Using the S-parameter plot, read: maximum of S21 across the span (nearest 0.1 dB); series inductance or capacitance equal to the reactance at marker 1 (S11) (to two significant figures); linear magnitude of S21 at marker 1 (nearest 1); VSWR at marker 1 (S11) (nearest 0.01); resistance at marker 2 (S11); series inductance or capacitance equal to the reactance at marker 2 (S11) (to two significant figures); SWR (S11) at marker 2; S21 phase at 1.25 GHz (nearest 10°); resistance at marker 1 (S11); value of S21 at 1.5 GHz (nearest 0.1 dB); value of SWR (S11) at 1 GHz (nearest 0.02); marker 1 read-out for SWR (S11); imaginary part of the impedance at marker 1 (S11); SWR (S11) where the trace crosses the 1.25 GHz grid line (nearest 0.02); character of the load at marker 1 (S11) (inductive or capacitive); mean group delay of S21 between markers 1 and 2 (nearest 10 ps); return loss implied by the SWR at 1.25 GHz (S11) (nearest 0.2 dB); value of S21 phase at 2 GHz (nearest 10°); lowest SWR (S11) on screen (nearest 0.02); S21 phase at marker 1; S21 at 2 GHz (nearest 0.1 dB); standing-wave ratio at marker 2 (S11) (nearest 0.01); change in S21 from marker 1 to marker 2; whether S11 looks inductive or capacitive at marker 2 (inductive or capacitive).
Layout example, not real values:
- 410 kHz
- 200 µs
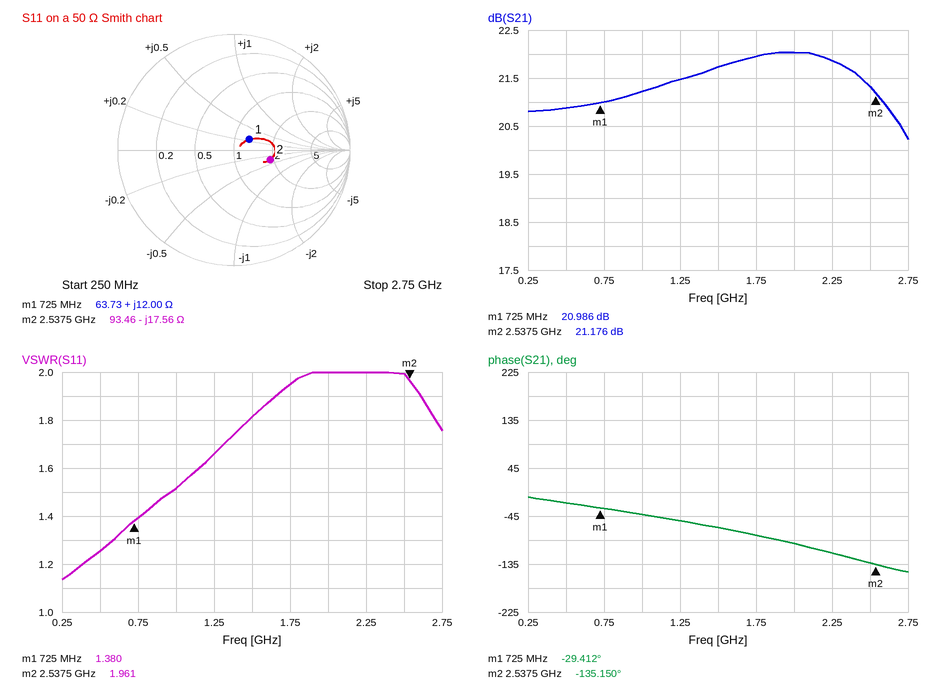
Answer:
- 22.0 dB
- 2.6 nH
- 11
- 1.38
- 93.46 Ω
- 3.6 pF
- 1.961
- -50°
- 63.73 Ω
- 21.7 dB
- 1.52
- 1.380
- +12.00 Ω
- 1.66
- inductive
- 160 ps
- 12.2 dB
- -100°
- 1.14
- -29.412°
- 22.0 dB
- 1.96
- 0.190 dB
- capacitive
